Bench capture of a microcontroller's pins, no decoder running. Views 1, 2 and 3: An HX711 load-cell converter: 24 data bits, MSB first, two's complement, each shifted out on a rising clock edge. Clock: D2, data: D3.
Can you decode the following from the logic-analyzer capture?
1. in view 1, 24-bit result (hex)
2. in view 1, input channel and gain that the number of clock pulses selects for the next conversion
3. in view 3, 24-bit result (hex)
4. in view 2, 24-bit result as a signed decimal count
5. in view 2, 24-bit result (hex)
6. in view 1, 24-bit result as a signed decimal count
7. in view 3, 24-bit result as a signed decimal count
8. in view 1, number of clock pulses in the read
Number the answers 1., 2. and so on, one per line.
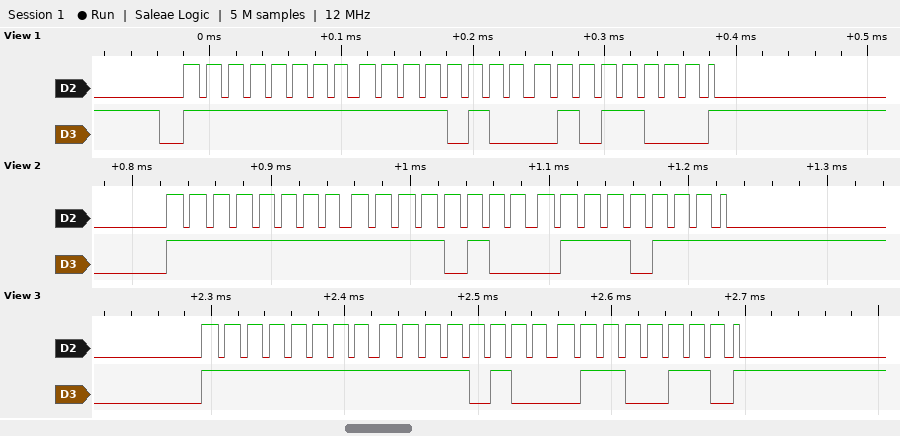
1. 0xFFF458
2. channel A, gain 128
3. 0xFFF466
4. -2953
5. 0xFFF477
6. -2984
7. -2970
8. 25
